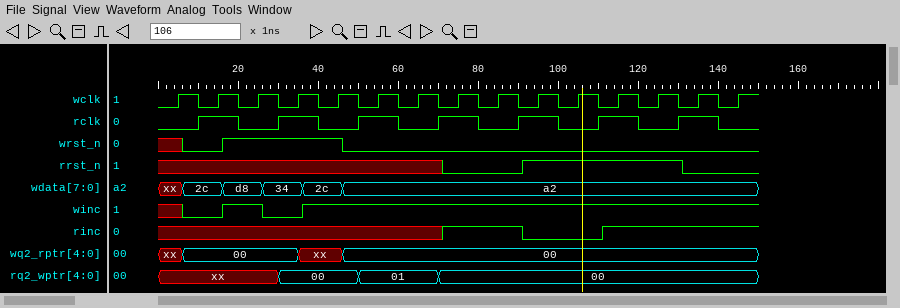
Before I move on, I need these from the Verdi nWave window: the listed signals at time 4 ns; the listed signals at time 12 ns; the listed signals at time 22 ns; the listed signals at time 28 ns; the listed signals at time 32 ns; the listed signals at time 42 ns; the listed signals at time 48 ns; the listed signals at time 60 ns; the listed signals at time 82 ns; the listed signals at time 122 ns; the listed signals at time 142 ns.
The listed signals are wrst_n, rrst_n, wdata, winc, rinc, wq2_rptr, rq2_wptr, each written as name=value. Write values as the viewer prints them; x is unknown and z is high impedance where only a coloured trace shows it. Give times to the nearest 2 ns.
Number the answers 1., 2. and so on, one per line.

1. wrst_n=x, rrst_n=x, wdata=xx, winc=x, rinc=x, wq2_rptr=xx, rq2_wptr=xx
2. wrst_n=0, rrst_n=x, wdata=2c, winc=0, rinc=x, wq2_rptr=00, rq2_wptr=xx
3. wrst_n=1, rrst_n=x, wdata=d8, winc=1, rinc=x, wq2_rptr=00, rq2_wptr=xx
4. wrst_n=1, rrst_n=x, wdata=34, winc=0, rinc=x, wq2_rptr=00, rq2_wptr=xx
5. wrst_n=1, rrst_n=x, wdata=34, winc=0, rinc=x, wq2_rptr=00, rq2_wptr=00
6. wrst_n=1, rrst_n=x, wdata=2c, winc=1, rinc=x, wq2_rptr=xx, rq2_wptr=00
7. wrst_n=0, rrst_n=x, wdata=a2, winc=1, rinc=x, wq2_rptr=00, rq2_wptr=00
8. wrst_n=0, rrst_n=x, wdata=a2, winc=1, rinc=x, wq2_rptr=00, rq2_wptr=01
9. wrst_n=0, rrst_n=0, wdata=a2, winc=1, rinc=1, wq2_rptr=00, rq2_wptr=00
10. wrst_n=0, rrst_n=1, wdata=a2, winc=1, rinc=1, wq2_rptr=00, rq2_wptr=00
11. wrst_n=0, rrst_n=0, wdata=a2, winc=1, rinc=1, wq2_rptr=00, rq2_wptr=00
